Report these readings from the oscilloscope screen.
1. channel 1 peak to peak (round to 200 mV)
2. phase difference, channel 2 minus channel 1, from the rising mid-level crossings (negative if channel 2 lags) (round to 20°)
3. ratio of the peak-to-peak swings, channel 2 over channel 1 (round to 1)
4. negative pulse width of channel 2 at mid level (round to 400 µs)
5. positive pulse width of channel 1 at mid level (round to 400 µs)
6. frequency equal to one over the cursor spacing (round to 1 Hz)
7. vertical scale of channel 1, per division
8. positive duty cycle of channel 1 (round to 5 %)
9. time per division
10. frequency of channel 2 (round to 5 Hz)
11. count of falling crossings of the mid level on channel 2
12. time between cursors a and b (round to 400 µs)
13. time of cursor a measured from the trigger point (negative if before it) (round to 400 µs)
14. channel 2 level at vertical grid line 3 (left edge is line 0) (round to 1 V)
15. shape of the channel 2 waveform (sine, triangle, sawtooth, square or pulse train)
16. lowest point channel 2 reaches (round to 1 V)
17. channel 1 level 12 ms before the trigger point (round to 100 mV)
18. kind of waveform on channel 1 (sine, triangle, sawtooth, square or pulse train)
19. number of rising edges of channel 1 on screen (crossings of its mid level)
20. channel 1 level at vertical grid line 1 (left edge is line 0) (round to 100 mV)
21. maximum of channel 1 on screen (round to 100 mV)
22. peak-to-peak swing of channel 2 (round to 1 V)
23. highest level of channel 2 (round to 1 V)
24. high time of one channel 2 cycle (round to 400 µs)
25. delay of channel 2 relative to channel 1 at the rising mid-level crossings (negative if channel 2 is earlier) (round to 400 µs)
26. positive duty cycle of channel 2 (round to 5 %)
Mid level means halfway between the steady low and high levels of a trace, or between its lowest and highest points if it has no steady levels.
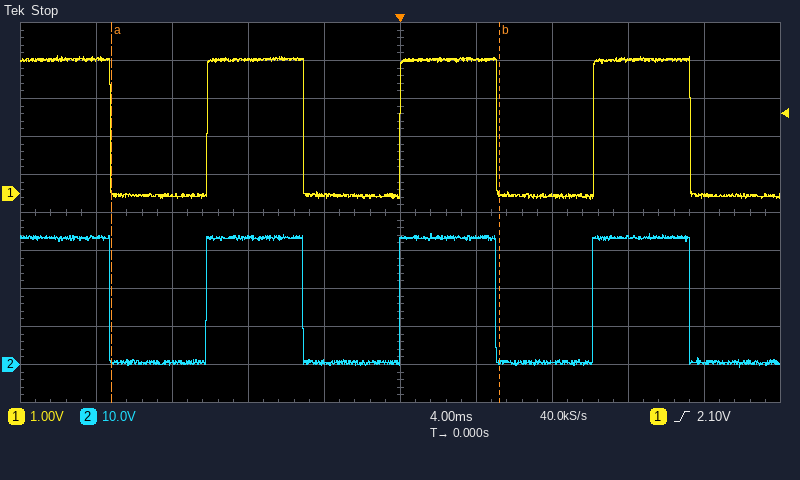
3.8 V
0°
9
5.2 ms
5.2 ms
49 Hz
1 V
50 %
4 ms
100 Hz
4
20.4 ms
-15.2 ms
33 V
square
-1 V
0.0 V
square
3
3.5 V
3.6 V
35 V
34 V
5.2 ms
0.0 ms
50 %
